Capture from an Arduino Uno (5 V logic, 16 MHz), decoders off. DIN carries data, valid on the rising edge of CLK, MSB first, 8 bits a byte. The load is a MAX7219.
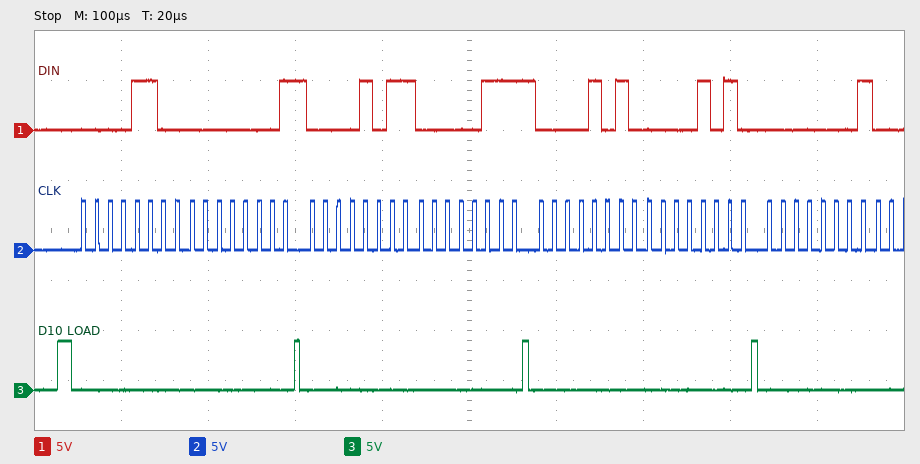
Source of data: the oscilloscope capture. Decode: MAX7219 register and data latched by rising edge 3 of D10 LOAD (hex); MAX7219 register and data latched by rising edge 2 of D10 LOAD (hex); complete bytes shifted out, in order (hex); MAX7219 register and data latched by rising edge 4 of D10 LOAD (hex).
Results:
register 0xB, data 0x07
register 0xC, data 0x01
0C 01 0B 07 0A 0A 01
register 0xA, data 0x0A
